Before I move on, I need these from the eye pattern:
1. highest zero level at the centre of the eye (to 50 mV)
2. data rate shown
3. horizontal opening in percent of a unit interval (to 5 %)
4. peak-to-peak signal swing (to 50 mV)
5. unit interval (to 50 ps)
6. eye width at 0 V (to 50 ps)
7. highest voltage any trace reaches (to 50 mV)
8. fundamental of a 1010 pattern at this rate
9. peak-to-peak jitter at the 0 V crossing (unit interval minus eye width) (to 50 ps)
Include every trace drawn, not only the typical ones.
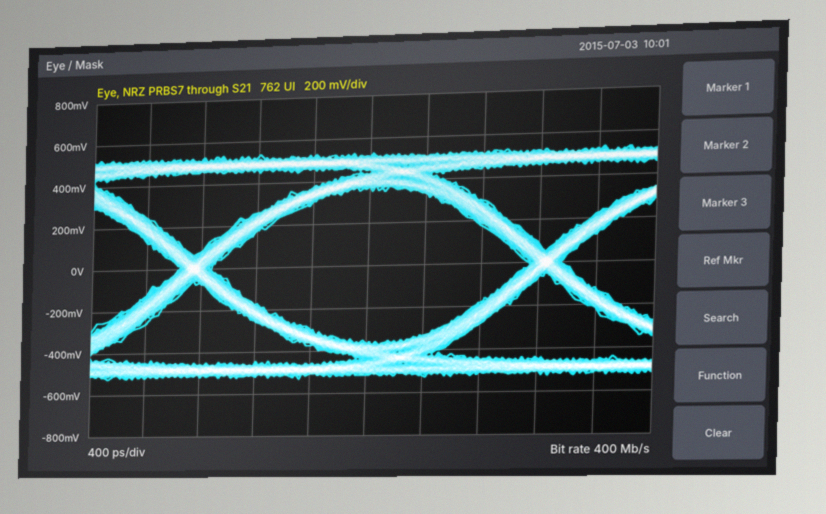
-350 mV
400 Mb/s
90 %
1.05 V
2.50 ns
2.25 ns
550 mV
200 MHz
250 ps
